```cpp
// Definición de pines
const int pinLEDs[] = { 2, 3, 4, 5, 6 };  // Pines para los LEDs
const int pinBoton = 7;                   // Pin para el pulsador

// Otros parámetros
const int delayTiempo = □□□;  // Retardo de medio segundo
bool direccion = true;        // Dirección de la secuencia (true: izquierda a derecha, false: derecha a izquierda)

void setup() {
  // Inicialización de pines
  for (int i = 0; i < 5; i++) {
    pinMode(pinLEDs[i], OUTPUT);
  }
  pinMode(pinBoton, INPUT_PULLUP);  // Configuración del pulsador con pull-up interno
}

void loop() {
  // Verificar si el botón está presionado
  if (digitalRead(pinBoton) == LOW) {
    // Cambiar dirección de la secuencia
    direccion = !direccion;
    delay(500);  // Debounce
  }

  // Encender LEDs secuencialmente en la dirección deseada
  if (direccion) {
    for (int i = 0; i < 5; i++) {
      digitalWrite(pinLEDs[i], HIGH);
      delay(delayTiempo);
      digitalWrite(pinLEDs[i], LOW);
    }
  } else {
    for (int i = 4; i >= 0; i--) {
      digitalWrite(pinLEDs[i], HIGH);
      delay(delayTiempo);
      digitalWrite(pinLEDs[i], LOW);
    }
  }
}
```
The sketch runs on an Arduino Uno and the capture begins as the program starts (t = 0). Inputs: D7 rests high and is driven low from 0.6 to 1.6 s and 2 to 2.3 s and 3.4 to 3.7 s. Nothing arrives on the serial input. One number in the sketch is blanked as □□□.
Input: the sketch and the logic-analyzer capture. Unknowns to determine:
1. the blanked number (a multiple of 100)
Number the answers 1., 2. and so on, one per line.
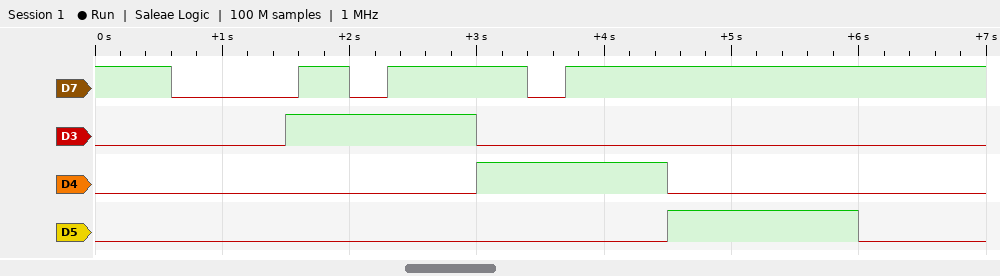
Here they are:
1. 1500
